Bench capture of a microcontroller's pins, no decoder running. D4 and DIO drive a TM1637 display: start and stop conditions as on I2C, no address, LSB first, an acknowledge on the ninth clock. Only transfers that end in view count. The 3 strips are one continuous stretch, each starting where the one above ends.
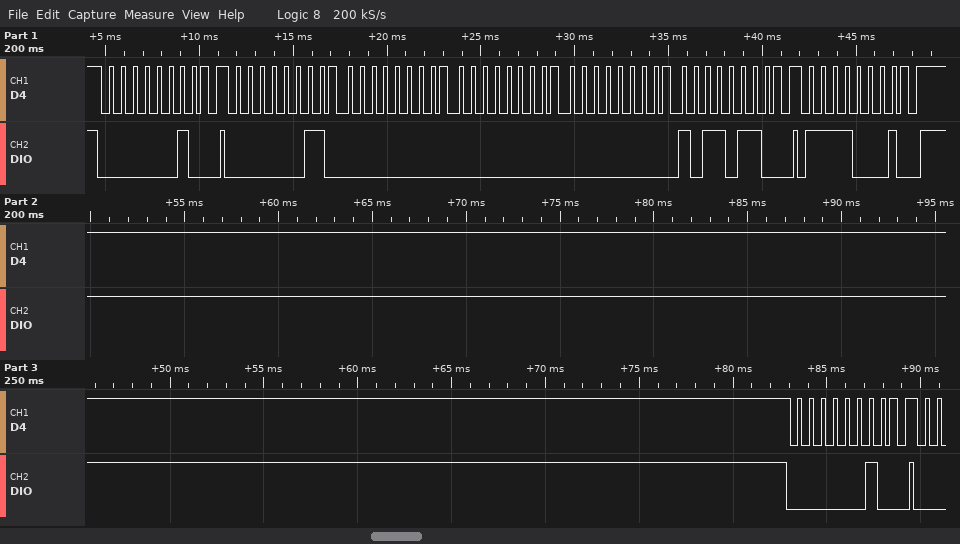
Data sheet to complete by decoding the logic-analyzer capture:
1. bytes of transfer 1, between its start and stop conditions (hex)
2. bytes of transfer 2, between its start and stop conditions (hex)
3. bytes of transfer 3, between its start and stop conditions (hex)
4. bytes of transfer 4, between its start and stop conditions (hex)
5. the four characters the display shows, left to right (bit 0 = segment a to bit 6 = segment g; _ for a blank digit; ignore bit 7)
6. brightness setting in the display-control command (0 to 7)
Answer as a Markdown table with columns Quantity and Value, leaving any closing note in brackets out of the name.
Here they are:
| Quantity | Value |
|---|---|
| bytes of transfer 1, between its start and stop conditions | 40 |
| bytes of transfer 2, between its start and stop conditions | C0 00 00 00 6D |
| bytes of transfer 3, between its start and stop conditions | 8F |
| bytes of transfer 4, between its start and stop conditions | 40 |
| the four characters the display shows, left to right | ___5 |
| brightness setting in the display-control command | 7 |
